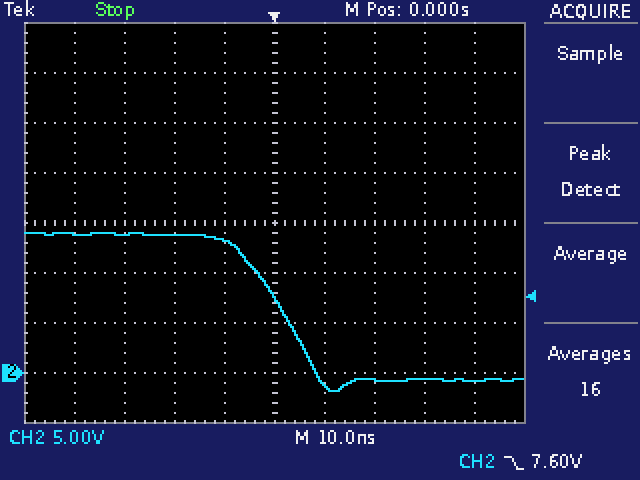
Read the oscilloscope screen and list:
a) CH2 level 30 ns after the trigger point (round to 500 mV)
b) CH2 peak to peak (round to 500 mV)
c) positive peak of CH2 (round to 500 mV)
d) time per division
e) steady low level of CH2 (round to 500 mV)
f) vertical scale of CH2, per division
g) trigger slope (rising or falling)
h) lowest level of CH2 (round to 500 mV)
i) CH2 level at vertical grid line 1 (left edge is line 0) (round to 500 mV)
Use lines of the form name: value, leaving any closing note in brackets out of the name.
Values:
CH2 level 30 ns after the trigger point: -500 mV
CH2 peak to peak: 16.0 V
positive peak of CH2: 14.0 V
time per division: 10 ns
steady low level of CH2: -500 mV
vertical scale of CH2, per division: 5 V
trigger slope: falling
lowest level of CH2: -2.0 V
CH2 level at vertical grid line 1 (left edge is line 0): 14.0 V
